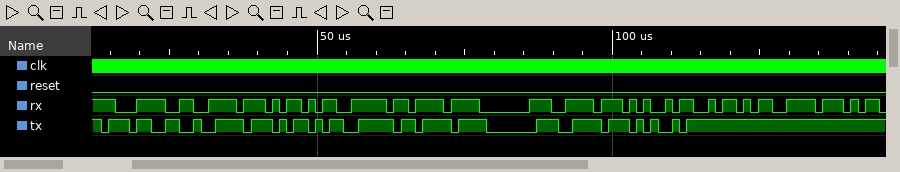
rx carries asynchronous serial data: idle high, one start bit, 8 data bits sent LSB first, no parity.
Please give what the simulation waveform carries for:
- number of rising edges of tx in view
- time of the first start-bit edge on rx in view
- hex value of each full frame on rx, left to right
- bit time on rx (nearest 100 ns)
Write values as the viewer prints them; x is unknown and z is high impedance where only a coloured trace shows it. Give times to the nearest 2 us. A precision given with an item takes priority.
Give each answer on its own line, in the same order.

21
16 us
3C, DE, AD, BE, EF, C0, DE, A5, 5A, DE
1200 ns
